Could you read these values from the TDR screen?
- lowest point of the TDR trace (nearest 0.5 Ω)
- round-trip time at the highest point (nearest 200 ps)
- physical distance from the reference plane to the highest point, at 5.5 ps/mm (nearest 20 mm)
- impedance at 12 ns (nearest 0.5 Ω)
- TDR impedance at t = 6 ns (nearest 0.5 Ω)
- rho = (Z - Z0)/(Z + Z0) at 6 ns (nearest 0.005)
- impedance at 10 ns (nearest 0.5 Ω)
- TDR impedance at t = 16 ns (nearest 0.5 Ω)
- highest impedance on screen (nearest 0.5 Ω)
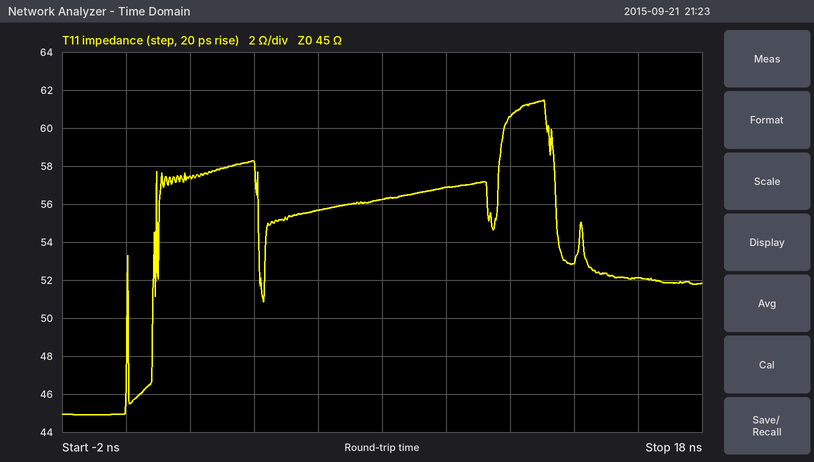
45.0 Ω
13.0 ns
1.18 m
60.5 Ω
55.5 Ω
+0.105
57.0 Ω
52.0 Ω
61.5 Ω
